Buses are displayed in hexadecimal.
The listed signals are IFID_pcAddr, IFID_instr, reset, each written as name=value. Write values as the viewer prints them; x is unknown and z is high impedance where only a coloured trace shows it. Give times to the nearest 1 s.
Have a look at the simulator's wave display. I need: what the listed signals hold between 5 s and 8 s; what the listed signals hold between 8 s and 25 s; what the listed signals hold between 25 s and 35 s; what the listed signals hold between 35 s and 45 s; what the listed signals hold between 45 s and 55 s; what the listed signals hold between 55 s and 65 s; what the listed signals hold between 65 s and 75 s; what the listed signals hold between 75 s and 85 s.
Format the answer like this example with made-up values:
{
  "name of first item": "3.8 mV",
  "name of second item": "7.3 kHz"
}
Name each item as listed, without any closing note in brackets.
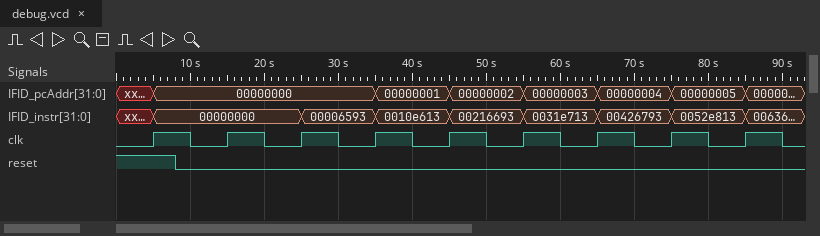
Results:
{
  "what the listed signals hold between 5 s and 8 s": "IFID_pcAddr=00000000, IFID_instr=00000000, reset=1",
  "what the listed signals hold between 8 s and 25 s": "IFID_pcAddr=00000000, IFID_instr=00000000, reset=0",
  "what the listed signals hold between 25 s and 35 s": "IFID_pcAddr=00000000, IFID_instr=00006593, reset=0",
  "what the listed signals hold between 35 s and 45 s": "IFID_pcAddr=00000001, IFID_instr=0010e613, reset=0",
  "what the listed signals hold between 45 s and 55 s": "IFID_pcAddr=00000002, IFID_instr=00216693, reset=0",
  "what the listed signals hold between 55 s and 65 s": "IFID_pcAddr=00000003, IFID_instr=0031e713, reset=0",
  "what the listed signals hold between 65 s and 75 s": "IFID_pcAddr=00000004, IFID_instr=00426793, reset=0",
  "what the listed signals hold between 75 s and 85 s": "IFID_pcAddr=00000005, IFID_instr=0052e813, reset=0"
}
